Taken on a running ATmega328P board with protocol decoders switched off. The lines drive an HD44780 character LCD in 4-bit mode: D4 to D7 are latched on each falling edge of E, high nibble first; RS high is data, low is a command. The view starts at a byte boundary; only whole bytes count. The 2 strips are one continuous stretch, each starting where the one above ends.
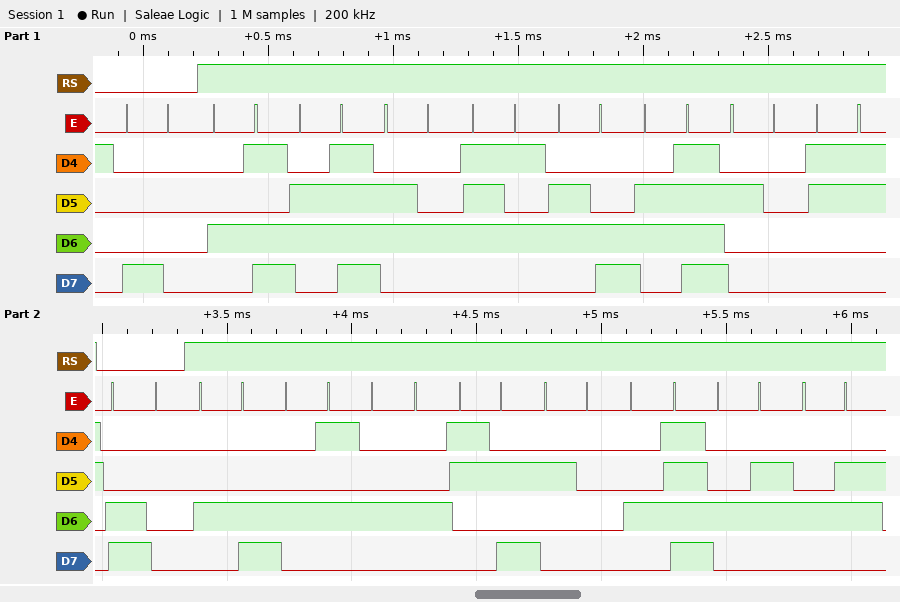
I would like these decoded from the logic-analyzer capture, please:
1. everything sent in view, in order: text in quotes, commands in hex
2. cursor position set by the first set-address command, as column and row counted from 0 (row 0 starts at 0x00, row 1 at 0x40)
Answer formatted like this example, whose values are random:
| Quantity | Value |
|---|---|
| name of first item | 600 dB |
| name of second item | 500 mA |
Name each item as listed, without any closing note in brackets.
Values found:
| Quantity | Value |
|---|---|
| everything sent in view, in order: text in quotes, commands in hex | 0x80 "Modulo 3" 0xC0 "LED: OFF" |
| cursor position set by the first set-address command, as column and row counted from 0 | column 0, row 0 |
